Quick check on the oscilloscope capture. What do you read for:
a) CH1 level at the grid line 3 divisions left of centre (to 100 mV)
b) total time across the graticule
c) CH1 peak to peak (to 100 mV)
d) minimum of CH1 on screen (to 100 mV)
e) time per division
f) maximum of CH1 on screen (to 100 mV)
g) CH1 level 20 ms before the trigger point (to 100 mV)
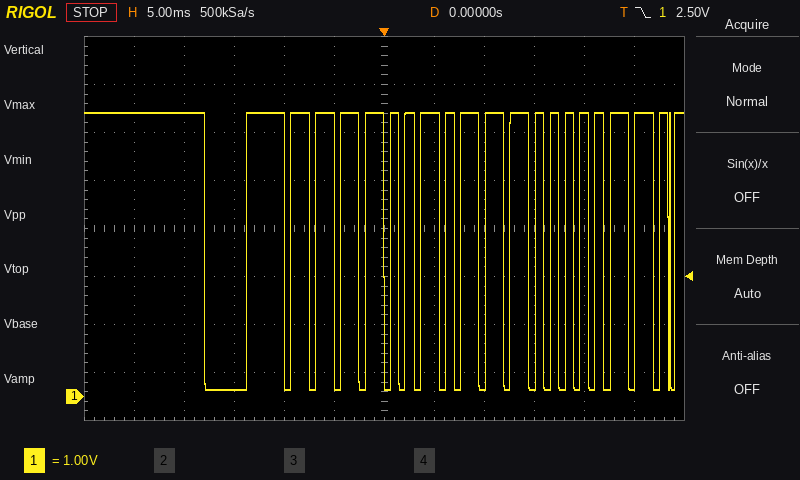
100 mV
60 ms
5.8 V
100 mV
5 ms
5.9 V
5.9 V
